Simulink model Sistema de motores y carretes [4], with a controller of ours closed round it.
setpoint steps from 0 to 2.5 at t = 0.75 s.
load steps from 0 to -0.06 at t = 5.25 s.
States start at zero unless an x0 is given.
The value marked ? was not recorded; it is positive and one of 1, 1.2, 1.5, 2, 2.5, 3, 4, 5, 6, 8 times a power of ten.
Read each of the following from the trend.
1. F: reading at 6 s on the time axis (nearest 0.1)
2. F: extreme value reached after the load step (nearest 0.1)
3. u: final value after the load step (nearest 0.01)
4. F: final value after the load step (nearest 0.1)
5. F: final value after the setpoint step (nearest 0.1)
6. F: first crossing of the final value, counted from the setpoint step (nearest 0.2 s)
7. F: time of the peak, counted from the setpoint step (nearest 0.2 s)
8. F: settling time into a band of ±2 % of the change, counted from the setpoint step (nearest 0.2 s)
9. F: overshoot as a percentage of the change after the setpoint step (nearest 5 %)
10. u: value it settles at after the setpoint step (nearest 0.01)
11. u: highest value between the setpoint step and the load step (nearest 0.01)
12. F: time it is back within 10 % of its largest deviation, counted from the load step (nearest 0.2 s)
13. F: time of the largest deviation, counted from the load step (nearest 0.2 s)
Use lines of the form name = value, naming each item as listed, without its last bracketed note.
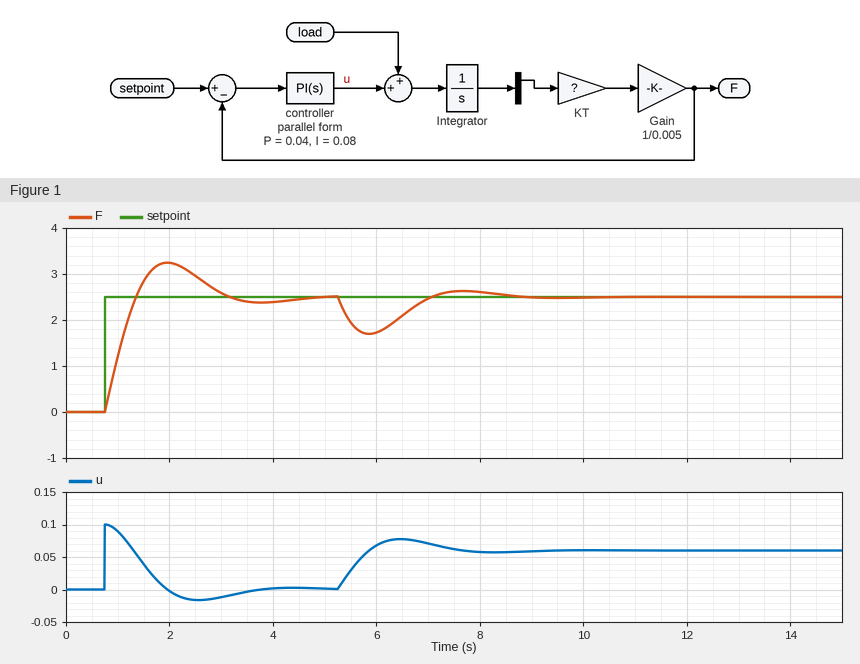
F: reading at 6 s on the time axis = 1.7
F: extreme value reached after the load step = 1.7
u: final value after the load step = 0.06
F: final value after the load step = 2.5
F: final value after the setpoint step = 2.5
F: first crossing of the final value, counted from the setpoint step = 0.6 s
F: time of the peak, counted from the setpoint step = 1.2 s
F: settling time into a band of ±2 % of the change, counted from the setpoint step = 3.8 s
F: overshoot as a percentage of the change after the setpoint step = 30 %
u: value it settles at after the setpoint step = 0.00
u: highest value between the setpoint step and the load step = 0.10
F: time it is back within 10 % of its largest deviation, counted from the load step = 3.0 s
F: time of the largest deviation, counted from the load step = 0.6 s
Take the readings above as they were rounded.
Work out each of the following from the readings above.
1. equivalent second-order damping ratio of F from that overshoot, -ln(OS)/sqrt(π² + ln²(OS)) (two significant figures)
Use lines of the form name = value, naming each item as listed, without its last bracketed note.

equivalent second-order damping ratio of F from that overshoot, -ln(OS)/sqrt(π² + ln²(OS)) = 0.36
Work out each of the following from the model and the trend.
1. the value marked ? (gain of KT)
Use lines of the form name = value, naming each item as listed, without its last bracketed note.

the value marked ? = 0.25
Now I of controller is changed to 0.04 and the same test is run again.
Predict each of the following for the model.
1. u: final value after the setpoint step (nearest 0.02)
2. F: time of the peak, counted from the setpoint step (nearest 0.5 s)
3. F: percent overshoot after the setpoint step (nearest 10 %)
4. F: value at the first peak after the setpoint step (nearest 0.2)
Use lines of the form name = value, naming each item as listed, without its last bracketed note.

u: final value after the setpoint step = 0.00
F: time of the peak, counted from the setpoint step = 1.5 s
F: percent overshoot after the setpoint step = 20 %
F: value at the first peak after the setpoint step = 3.0
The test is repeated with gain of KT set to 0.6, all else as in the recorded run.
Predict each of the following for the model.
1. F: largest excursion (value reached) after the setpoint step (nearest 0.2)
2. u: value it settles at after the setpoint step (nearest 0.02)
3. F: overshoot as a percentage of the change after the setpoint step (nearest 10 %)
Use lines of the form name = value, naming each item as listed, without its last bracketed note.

F: largest excursion (value reached) after the setpoint step = 3.0
u: value it settles at after the setpoint step = 0.00
F: overshoot as a percentage of the change after the setpoint step = 20 %
